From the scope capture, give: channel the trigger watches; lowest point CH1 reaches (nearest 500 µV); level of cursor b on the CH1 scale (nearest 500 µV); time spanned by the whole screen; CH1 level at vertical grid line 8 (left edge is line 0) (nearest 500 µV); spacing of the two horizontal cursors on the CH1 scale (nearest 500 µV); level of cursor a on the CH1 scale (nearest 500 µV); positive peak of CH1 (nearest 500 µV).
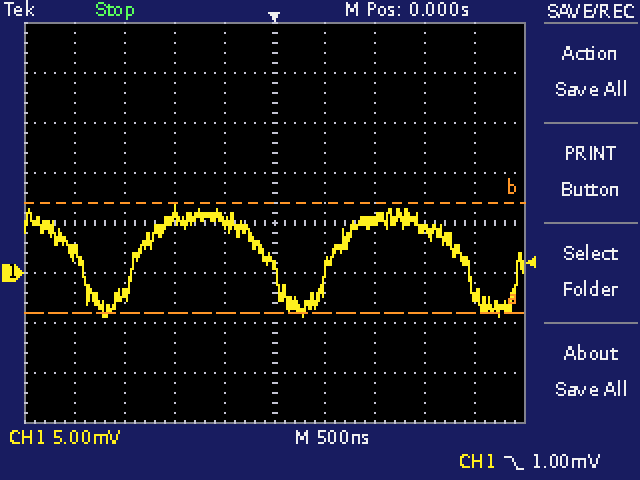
CH1
-4.5 mV
7.0 mV
5 µs
4.5 mV
11.0 mV
-4.0 mV
7.0 mV
